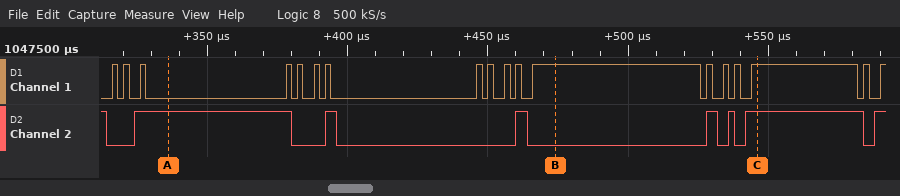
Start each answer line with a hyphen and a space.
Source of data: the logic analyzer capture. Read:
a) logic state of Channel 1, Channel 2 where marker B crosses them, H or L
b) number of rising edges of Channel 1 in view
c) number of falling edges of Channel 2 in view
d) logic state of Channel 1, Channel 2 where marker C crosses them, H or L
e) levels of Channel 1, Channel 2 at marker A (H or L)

- Channel 1=H, Channel 2=L
- 18
- 7
- Channel 1=H, Channel 2=H
- Channel 1=L, Channel 2=H
